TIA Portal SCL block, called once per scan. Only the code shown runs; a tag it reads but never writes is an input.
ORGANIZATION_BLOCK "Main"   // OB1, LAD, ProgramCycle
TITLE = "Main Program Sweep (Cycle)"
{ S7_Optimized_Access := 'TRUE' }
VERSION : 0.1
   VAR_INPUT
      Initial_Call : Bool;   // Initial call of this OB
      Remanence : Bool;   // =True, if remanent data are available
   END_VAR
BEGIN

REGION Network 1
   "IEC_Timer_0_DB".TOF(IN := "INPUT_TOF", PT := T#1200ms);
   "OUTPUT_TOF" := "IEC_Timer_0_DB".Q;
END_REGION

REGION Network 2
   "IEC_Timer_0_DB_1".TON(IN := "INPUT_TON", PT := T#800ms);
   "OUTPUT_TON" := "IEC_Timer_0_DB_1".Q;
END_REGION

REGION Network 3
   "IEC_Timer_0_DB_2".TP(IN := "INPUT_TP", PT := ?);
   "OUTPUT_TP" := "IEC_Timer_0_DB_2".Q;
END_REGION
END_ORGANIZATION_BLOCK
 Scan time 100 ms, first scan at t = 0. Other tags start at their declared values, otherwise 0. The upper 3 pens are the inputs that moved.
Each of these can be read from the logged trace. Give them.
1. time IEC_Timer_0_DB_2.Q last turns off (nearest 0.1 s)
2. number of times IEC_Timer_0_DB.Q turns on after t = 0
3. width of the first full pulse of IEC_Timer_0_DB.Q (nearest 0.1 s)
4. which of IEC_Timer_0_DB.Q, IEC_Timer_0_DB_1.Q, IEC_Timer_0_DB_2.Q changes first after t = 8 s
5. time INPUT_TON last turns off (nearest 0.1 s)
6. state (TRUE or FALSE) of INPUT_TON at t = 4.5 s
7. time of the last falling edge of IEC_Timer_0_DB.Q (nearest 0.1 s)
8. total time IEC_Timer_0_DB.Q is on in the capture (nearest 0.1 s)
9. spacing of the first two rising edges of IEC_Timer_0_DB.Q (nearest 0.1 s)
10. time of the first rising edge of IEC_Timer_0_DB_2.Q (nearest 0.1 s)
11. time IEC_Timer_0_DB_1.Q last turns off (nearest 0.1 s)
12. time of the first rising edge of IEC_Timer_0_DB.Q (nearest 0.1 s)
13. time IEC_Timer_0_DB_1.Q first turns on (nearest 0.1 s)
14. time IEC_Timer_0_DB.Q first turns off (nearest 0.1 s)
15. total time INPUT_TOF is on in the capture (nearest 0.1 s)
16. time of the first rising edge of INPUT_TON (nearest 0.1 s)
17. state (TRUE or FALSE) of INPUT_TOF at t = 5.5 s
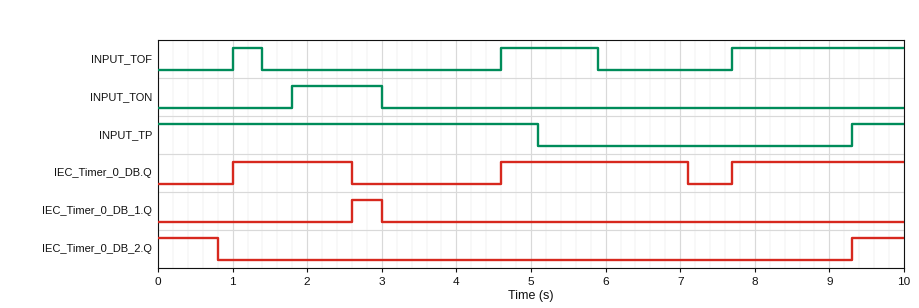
0.8 s
3
1.6 s
IEC_Timer_0_DB_2.Q
3.0 s
FALSE
7.1 s
6.4 s
3.6 s
9.3 s
3.0 s
1.0 s
2.6 s
2.6 s
4.0 s
1.8 s
TRUE
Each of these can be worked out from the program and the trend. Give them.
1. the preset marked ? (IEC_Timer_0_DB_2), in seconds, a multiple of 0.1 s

0.8 s
